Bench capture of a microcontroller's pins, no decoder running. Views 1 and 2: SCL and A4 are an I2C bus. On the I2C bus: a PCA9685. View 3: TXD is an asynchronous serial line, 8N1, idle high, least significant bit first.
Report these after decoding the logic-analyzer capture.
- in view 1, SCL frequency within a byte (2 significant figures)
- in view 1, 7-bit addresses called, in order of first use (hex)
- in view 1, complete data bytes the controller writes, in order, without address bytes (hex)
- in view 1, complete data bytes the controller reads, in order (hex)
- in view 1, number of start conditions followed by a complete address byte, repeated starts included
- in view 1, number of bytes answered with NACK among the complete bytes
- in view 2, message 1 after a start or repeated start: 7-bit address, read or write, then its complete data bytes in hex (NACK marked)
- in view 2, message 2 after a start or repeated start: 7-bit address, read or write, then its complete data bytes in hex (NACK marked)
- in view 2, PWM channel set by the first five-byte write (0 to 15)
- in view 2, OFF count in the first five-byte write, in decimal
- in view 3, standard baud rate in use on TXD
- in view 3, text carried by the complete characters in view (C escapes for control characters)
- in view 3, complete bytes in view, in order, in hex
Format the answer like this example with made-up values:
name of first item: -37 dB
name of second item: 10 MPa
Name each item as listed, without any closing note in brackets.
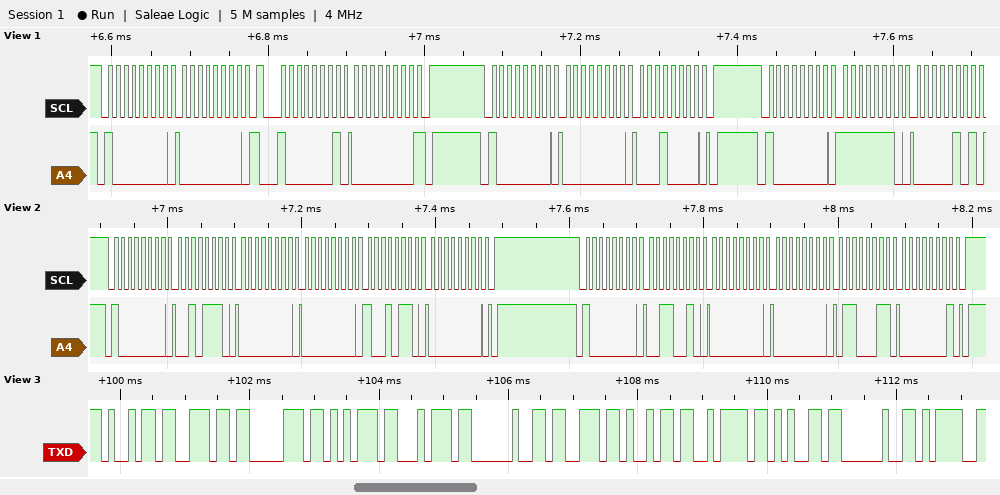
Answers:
in view 1, SCL frequency within a byte: 100 kHz
in view 1, 7-bit addresses called, in order of first use: 0x40
in view 1, complete data bytes the controller writes, in order, without address bytes: 00 00 10 FE 05
in view 1, complete data bytes the controller reads, in order: 00
in view 1, number of start conditions followed by a complete address byte, repeated starts included: 4
in view 1, number of bytes answered with NACK among the complete bytes: 1
in view 2, message 1 after a start or repeated start: 7-bit address, read or write, then its complete data bytes in hex: 0x40 write: 2E 00 00 96 00
in view 2, message 2 after a start or repeated start: 7-bit address, read or write, then its complete data bytes in hex: 0x40 write: 32 00 00 63 01
in view 2, PWM channel set by the first five-byte write: 10
in view 2, OFF count in the first five-byte write, in decimal: 150
in view 3, standard baud rate in use on TXD: 9600 baud
in view 3, text carried by the complete characters in view: "input size ="
in view 3, complete bytes in view, in order, in hex: 69 6E 70 75 74 20 73 69 7A 65 20 3D
